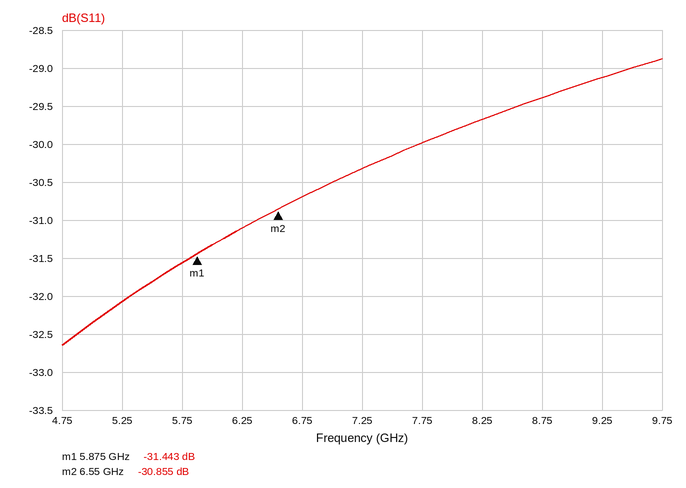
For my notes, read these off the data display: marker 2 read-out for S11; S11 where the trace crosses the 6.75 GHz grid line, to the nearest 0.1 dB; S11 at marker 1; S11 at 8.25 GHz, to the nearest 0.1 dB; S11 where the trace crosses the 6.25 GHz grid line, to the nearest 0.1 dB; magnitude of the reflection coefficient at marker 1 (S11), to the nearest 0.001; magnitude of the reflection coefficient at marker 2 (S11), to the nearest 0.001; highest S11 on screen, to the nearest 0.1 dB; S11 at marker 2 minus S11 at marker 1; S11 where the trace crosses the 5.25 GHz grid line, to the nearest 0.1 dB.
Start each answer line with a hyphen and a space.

- -30.855 dB
- -30.7 dB
- -31.443 dB
- -29.7 dB
- -31.1 dB
- 0.027
- 0.029
- -28.9 dB
- 0.588 dB
- -32.1 dB
